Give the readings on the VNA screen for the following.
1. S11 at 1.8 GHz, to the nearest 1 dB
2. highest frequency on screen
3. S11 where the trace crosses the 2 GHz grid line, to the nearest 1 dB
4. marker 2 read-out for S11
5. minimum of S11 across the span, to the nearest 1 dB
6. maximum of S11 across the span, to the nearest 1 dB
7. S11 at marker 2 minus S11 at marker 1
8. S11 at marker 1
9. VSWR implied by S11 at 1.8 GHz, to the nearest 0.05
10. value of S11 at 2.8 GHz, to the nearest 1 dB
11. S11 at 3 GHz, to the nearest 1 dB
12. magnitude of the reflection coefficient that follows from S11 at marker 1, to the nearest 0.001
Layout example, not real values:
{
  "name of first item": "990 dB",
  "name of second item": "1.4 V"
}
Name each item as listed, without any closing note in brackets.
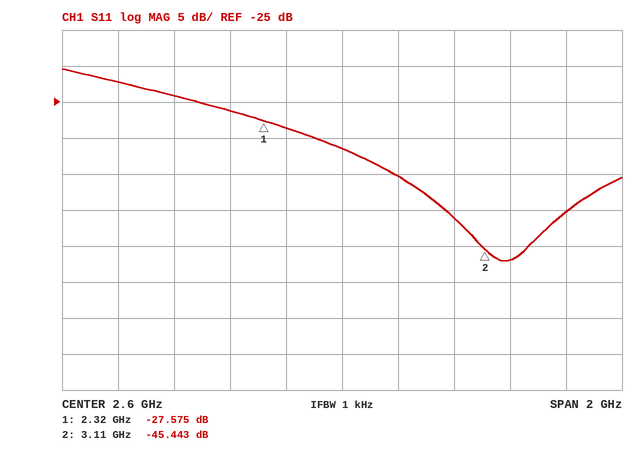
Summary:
{
  "S11 at 1.8 GHz, to the nearest 1 dB": "-22 dB",
  "highest frequency on screen": "3.6 GHz",
  "S11 where the trace crosses the 2 GHz grid line, to the nearest 1 dB": "-24 dB",
  "marker 2 read-out for S11": "-45.443 dB",
  "minimum of S11 across the span, to the nearest 1 dB": "-47 dB",
  "maximum of S11 across the span, to the nearest 1 dB": "-20 dB",
  "S11 at marker 2 minus S11 at marker 1": "-17.868 dB",
  "S11 at marker 1": "-27.575 dB",
  "VSWR implied by S11 at 1.8 GHz, to the nearest 0.05": "1.15",
  "value of S11 at 2.8 GHz, to the nearest 1 dB": "-35 dB",
  "S11 at 3 GHz, to the nearest 1 dB": "-41 dB",
  "magnitude of the reflection coefficient that follows from S11 at marker 1, to the nearest 0.001": "0.042"
}
